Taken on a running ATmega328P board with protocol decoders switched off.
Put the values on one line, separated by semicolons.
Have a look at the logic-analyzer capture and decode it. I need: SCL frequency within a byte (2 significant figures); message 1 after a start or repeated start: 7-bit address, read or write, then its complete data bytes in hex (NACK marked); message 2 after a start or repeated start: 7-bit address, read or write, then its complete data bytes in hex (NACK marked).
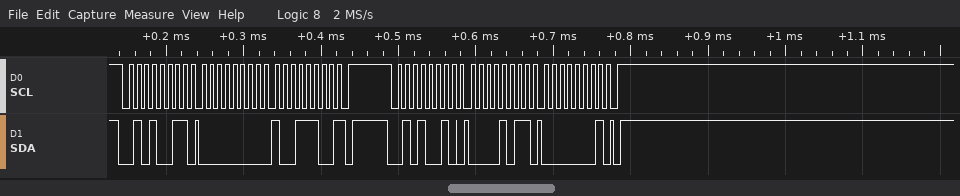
100 kHz; 0x29 read: 00 9C NACK; 0x29 write: 0B 01
